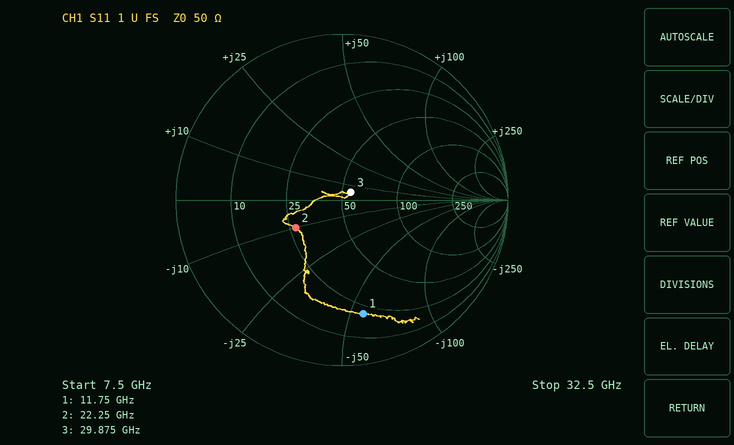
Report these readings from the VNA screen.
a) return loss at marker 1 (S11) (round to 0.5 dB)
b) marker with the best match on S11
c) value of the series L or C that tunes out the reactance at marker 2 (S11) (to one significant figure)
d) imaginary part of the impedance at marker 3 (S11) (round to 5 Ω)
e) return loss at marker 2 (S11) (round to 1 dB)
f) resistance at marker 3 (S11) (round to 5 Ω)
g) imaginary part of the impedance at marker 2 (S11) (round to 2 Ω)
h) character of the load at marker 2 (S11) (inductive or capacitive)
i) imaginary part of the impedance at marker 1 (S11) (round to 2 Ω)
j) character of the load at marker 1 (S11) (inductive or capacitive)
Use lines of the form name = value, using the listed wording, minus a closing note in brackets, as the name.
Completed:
return loss at marker 1 (S11) = 3.0 dB
marker with the best match on S11 = marker 3
value of the series L or C that tunes out the reactance at marker 2 (S11) = 70 pH
imaginary part of the impedance at marker 3 (S11) = +5 Ω
return loss at marker 2 (S11) = 10 dB
resistance at marker 3 (S11) = 55 Ω
imaginary part of the impedance at marker 2 (S11) = -10 Ω
character of the load at marker 2 (S11) = capacitive
imaginary part of the impedance at marker 1 (S11) = -56 Ω
character of the load at marker 1 (S11) = capacitive
